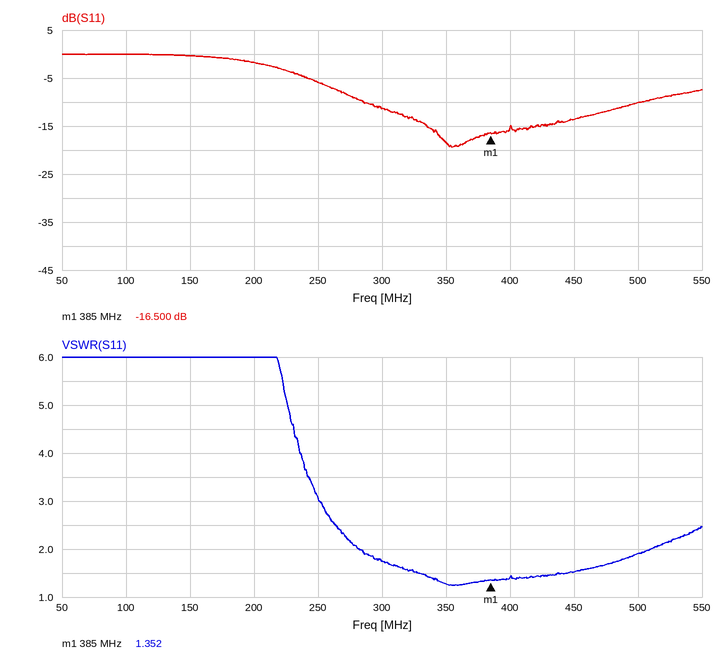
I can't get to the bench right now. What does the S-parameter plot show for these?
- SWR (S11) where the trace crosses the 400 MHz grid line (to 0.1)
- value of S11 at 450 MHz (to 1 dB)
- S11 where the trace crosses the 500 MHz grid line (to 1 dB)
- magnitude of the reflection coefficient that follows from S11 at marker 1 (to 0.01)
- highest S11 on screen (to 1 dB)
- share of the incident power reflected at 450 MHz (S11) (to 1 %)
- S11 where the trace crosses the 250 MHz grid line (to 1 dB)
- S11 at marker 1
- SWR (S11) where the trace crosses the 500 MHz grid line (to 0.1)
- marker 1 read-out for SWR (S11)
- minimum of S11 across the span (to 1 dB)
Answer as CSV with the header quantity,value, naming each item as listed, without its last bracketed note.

quantity,value
SWR (S11) where the trace crosses the 400 MHz grid line,1.4
value of S11 at 450 MHz,-14 dB
S11 where the trace crosses the 500 MHz grid line,-10 dB
magnitude of the reflection coefficient that follows from S11 at marker 1,0.15
highest S11 on screen,0 dB
share of the incident power reflected at 450 MHz (S11),4 %
S11 where the trace crosses the 250 MHz grid line,-6 dB
S11 at marker 1,-16.500 dB
SWR (S11) where the trace crosses the 500 MHz grid line,1.9
marker 1 read-out for SWR,1.352
minimum of S11 across the span,-19 dB
